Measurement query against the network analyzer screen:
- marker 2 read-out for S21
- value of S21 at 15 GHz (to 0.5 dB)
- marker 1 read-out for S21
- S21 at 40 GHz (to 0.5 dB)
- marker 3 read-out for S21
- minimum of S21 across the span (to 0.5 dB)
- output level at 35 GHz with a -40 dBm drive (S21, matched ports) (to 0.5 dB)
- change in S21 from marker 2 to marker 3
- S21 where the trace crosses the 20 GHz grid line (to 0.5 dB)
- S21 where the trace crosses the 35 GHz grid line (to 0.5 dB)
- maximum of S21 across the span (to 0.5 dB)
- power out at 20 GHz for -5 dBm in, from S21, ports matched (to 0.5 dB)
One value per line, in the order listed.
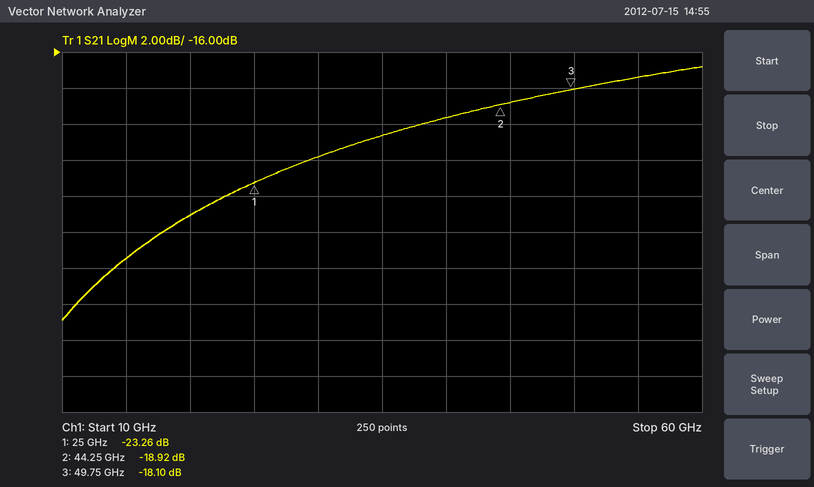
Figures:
-18.92 dB
-27.5 dB
-23.26 dB
-19.5 dB
-18.10 dB
-31.0 dB
-60.5 dBm
0.82 dB
-25.0 dB
-20.5 dB
-17.0 dB
-30.0 dBm
